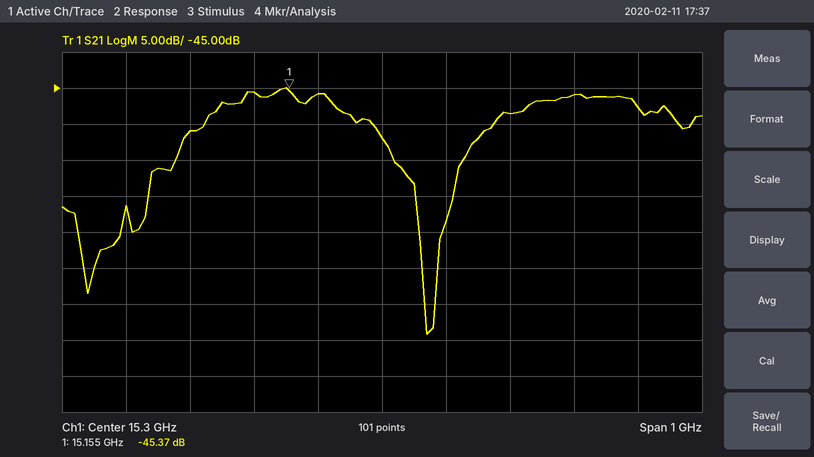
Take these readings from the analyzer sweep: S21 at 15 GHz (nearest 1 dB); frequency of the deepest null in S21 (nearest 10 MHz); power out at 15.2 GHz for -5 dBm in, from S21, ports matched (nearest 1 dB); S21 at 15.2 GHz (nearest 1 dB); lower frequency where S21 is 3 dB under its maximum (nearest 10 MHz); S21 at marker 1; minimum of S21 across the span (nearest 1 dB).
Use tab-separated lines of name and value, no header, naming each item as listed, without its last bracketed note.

S21 at 15 GHz	-51 dB
frequency of the deepest null in S21	15.37 GHz
power out at 15.2 GHz for -5 dBm in, from S21, ports matched	-51 dBm
S21 at 15.2 GHz	-46 dB
lower frequency where S21 is 3 dB under its maximum	15.04 GHz
S21 at marker 1	-45.37 dB
minimum of S21 across the span	-79 dB
